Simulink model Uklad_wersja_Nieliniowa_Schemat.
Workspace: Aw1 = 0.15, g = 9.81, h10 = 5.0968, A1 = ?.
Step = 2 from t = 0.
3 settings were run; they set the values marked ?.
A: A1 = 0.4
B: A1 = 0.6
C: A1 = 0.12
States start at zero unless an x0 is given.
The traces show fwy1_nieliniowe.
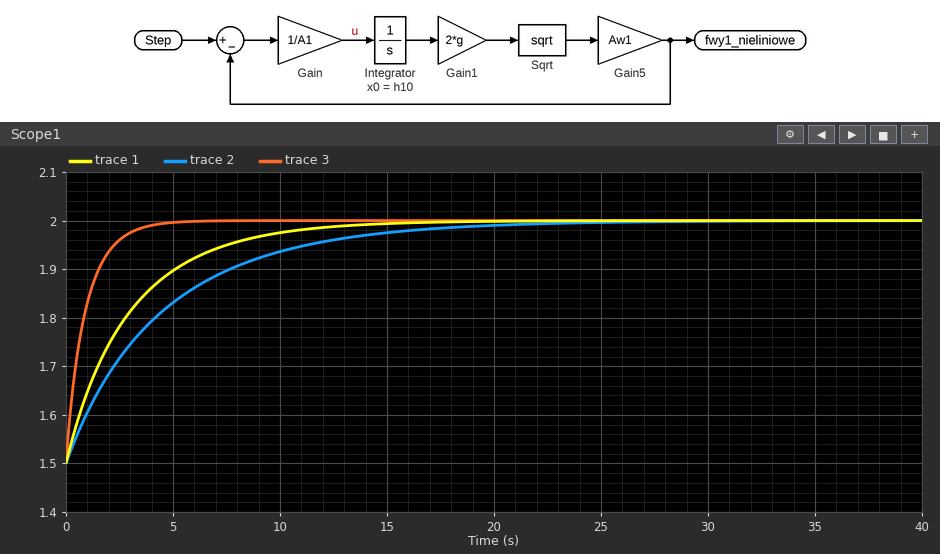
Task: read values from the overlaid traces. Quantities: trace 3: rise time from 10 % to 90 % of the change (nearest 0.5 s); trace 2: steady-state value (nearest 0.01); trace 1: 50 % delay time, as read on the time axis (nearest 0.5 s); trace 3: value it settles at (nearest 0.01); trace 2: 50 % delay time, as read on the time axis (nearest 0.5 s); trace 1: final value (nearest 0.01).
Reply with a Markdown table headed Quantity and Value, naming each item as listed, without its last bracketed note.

| Quantity | Value |
|---|---|
| trace 3: rise time from 10 % to 90 % of the change | 2.0 s |
| trace 2: steady-state value | 2.00 |
| trace 1: 50 % delay time, as read on the time axis | 2.0 s |
| trace 3: value it settles at | 2.00 |
| trace 2: 50 % delay time, as read on the time axis | 3.0 s |
| trace 1: final value | 2.00 |
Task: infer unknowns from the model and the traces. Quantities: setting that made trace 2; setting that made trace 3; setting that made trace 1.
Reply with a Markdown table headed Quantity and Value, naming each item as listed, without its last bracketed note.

| Quantity | Value |
|---|---|
| setting that made trace 2 | B |
| setting that made trace 3 | C |
| setting that made trace 1 | A |
